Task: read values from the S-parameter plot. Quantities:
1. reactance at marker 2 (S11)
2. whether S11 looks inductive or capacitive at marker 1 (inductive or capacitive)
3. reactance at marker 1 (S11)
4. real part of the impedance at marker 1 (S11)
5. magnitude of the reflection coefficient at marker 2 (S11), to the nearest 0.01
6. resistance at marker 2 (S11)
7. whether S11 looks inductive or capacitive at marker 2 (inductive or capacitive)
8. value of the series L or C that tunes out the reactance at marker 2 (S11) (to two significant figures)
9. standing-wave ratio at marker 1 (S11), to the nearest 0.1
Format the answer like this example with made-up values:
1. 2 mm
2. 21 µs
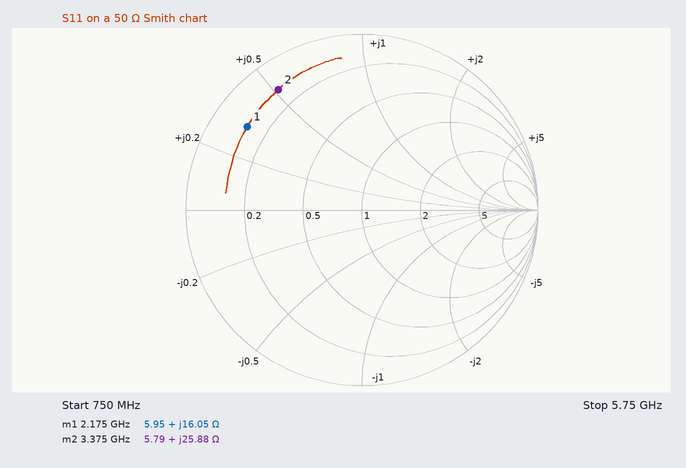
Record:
1. +25.88 Ω
2. inductive
3. +16.05 Ω
4. 5.95 Ω
5. 0.83
6. 5.79 Ω
7. inductive
8. 1.8 pF
9. 9.3
